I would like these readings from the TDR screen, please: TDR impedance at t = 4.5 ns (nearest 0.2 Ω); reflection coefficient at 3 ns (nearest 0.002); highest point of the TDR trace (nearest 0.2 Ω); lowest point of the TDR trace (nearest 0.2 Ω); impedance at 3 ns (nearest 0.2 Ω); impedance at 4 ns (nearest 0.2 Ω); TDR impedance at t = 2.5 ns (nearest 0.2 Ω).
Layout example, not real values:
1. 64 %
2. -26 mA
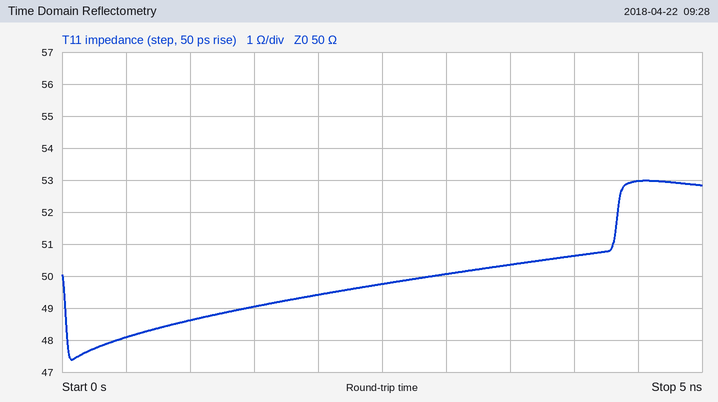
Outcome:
1. 53.0 Ω
2. 0.000
3. 53.0 Ω
4. 47.4 Ω
5. 50.0 Ω
6. 50.6 Ω
7. 49.8 Ω
